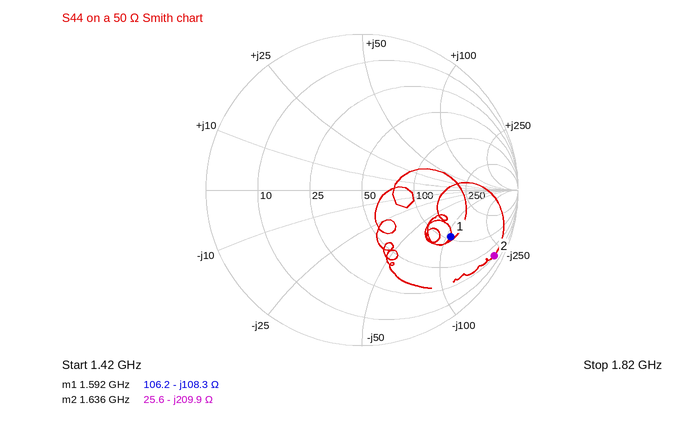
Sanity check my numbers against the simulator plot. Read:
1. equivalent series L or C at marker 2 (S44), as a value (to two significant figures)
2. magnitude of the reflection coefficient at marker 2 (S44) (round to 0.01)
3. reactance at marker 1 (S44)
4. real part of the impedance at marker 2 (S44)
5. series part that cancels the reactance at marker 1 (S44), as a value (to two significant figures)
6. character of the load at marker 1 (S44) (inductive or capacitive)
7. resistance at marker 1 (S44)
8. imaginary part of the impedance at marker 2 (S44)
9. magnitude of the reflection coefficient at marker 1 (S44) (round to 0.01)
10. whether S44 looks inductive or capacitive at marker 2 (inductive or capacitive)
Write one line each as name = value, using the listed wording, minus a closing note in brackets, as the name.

equivalent series L or C at marker 2 (S44), as a value = 460 fF
magnitude of the reflection coefficient at marker 2 (S44) = 0.95
reactance at marker 1 = -108.3 Ω
real part of the impedance at marker 2 = 25.6 Ω
series part that cancels the reactance at marker 1 (S44), as a value = 11 nH
character of the load at marker 1 (S44) = capacitive
resistance at marker 1 = 106.2 Ω
imaginary part of the impedance at marker 2 = -209.9 Ω
magnitude of the reflection coefficient at marker 1 (S44) = 0.64
whether S44 looks inductive or capacitive at marker 2 = capacitive
